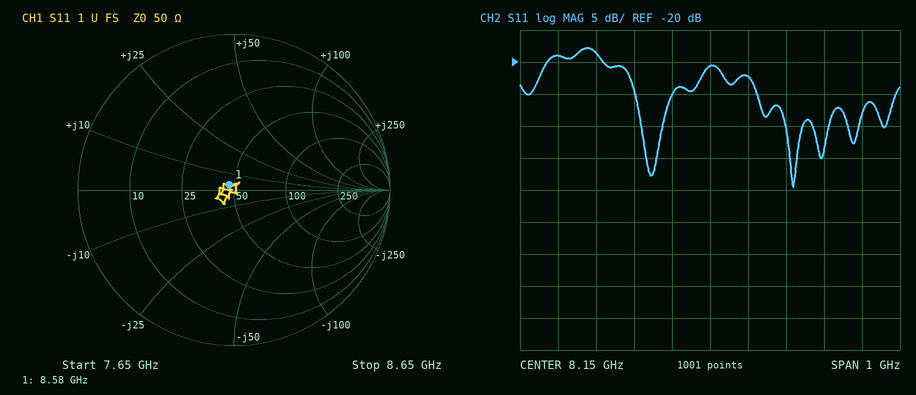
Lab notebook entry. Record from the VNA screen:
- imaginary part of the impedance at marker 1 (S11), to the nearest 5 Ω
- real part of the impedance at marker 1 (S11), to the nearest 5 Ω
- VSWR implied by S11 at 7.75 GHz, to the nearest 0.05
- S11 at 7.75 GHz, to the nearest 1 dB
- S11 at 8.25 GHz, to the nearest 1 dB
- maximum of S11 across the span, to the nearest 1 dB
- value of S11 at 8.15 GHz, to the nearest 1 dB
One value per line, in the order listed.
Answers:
+5 Ω
45 Ω
1.25
-19 dB
-22 dB
-18 dB
-21 dB
